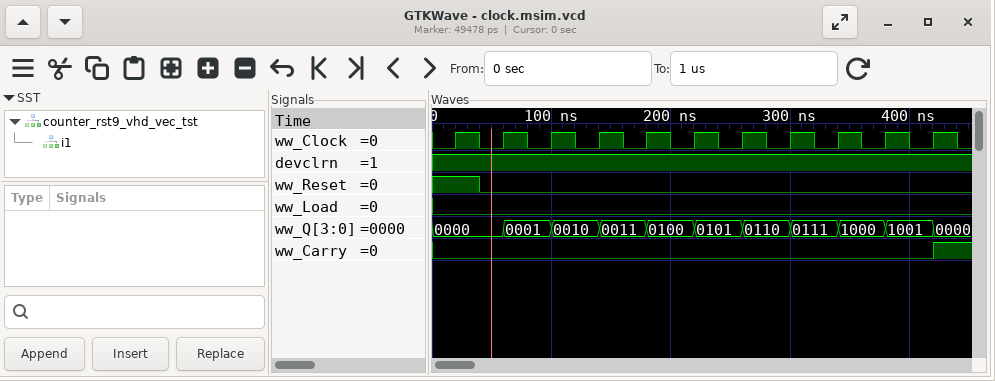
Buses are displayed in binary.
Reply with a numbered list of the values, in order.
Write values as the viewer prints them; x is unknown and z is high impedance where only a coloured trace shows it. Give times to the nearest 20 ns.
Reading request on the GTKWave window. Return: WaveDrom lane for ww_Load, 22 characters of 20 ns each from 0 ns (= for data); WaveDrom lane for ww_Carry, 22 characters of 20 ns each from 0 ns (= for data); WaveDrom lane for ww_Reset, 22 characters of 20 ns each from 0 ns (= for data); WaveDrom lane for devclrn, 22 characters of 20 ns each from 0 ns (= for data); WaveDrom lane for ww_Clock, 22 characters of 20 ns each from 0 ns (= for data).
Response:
1. {name: 'ww_Load', wave: '0.....................'}
2. {name: 'ww_Carry', wave: '0....................1'}
3. {name: 'ww_Reset', wave: '1.0...................'}
4. {name: 'devclrn', wave: '1.....................'}
5. {name: 'ww_Clock', wave: '0101010101010101010101'}
